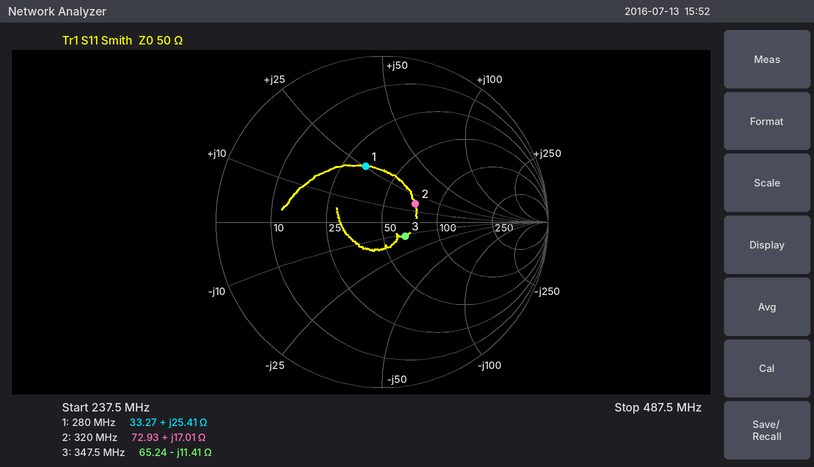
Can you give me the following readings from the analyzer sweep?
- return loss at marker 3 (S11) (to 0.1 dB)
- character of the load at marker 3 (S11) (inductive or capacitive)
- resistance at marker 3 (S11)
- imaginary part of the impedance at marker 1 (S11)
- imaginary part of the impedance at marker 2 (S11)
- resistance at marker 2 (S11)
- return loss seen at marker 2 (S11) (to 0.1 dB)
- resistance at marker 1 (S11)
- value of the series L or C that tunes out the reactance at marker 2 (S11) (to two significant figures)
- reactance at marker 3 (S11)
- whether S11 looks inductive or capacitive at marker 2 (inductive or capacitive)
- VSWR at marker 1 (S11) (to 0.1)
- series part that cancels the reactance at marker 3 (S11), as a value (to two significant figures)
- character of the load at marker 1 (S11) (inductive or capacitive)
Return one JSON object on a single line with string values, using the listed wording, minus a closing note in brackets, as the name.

{"return loss at marker 3 (S11)": "15.7 dB", "character of the load at marker 3 (S11)": "capacitive", "resistance at marker 3": "65.24 Ω", "imaginary part of the impedance at marker 1": "+25.41 Ω", "imaginary part of the impedance at marker 2": "+17.01 Ω", "resistance at marker 2": "72.93 Ω", "return loss seen at marker 2 (S11)": "12.8 dB", "resistance at marker 1": "33.27 Ω", "value of the series L or C that tunes out the reactance at marker 2 (S11)": "29 pF", "reactance at marker 3": "-11.41 Ω", "whether S11 looks inductive or capacitive at marker 2": "inductive", "VSWR at marker 1 (S11)": "2.1", "series part that cancels the reactance at marker 3 (S11), as a value": "5.2 nH", "character of the load at marker 1 (S11)": "inductive"}
